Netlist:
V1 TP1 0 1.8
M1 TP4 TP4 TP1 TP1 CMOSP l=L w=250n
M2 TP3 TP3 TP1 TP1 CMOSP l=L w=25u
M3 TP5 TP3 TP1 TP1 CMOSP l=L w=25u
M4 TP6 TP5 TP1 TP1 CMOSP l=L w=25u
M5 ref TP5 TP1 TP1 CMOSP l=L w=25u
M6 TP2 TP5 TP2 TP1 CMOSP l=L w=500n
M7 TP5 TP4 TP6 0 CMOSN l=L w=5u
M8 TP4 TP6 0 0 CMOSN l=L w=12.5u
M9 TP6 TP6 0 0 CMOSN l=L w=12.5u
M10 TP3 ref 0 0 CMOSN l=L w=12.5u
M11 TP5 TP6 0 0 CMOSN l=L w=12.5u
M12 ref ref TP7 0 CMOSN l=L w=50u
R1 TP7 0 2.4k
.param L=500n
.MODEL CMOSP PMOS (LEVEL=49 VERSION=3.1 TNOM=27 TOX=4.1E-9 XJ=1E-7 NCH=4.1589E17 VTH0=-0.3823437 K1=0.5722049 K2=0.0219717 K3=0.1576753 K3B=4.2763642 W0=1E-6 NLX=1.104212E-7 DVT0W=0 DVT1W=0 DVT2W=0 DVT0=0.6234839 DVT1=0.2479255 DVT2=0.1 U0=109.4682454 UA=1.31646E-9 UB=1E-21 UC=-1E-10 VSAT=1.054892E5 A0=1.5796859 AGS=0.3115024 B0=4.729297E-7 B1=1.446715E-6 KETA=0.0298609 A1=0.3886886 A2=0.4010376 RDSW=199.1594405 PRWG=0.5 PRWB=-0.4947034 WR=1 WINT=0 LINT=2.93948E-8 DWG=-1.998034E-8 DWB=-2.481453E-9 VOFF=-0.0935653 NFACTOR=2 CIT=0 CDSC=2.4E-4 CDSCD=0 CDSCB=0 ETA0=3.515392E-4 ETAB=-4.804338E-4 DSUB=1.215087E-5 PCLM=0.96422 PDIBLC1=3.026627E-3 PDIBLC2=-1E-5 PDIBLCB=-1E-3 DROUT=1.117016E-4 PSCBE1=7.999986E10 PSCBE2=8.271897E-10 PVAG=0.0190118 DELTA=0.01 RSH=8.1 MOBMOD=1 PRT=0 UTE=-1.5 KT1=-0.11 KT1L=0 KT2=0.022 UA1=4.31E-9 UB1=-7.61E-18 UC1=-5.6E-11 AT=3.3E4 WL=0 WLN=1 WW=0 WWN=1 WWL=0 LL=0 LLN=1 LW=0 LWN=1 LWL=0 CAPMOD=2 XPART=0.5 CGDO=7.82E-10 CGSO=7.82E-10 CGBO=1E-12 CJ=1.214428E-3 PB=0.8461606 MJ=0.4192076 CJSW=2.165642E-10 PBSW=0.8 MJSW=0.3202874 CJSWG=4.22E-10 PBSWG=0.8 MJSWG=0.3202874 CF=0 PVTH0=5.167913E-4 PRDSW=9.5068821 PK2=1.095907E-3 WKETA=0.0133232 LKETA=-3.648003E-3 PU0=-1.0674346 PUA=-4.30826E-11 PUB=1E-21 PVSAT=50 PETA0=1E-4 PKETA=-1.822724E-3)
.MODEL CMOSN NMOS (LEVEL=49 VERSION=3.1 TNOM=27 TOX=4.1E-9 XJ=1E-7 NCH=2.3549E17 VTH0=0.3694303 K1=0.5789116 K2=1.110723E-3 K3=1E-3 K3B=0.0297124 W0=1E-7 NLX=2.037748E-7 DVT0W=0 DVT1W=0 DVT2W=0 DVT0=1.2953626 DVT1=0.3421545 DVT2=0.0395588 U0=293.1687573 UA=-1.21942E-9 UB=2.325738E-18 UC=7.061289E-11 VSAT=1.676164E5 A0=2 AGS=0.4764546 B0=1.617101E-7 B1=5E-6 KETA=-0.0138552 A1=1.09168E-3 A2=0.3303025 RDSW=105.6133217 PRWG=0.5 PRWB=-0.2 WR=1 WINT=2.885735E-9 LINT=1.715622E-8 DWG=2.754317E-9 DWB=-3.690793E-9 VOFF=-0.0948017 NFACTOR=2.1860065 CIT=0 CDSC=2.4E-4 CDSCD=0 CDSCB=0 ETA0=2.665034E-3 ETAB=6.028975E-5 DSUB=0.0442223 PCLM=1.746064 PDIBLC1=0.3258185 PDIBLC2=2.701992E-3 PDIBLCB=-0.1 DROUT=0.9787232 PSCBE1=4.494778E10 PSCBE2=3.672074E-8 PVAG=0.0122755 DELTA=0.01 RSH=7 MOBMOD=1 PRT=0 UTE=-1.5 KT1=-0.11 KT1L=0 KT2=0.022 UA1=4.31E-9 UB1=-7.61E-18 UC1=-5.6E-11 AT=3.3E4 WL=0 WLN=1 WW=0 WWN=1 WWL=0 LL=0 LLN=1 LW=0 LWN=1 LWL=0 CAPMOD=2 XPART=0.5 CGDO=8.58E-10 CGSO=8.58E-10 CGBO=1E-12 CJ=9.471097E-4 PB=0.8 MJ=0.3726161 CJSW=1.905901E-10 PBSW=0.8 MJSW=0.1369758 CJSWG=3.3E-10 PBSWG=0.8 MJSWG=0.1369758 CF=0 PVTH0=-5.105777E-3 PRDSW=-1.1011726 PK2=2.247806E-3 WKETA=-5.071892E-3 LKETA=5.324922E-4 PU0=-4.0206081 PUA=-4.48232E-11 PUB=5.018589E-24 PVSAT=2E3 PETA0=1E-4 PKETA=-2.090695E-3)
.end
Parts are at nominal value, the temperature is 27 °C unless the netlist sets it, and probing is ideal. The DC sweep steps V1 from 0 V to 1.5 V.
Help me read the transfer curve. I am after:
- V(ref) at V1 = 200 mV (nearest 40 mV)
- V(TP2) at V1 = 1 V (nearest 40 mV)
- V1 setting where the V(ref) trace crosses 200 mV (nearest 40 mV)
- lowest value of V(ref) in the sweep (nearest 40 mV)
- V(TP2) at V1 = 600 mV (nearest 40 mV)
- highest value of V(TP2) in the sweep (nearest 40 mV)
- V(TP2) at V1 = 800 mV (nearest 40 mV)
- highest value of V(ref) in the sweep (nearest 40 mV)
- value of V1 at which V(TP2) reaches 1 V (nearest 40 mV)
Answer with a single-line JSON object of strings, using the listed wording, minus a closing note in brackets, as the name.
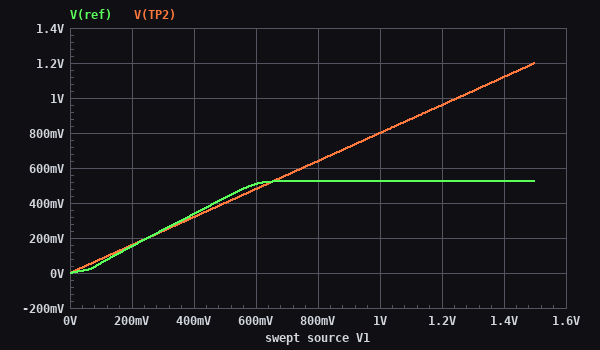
{"V(ref) at V1 = 200 mV": "160 mV", "V(TP2) at V1 = 1 V": "800 mV", "V1 setting where the V(ref) trace crosses 200 mV": "240 mV", "lowest value of V(ref) in the sweep": "0 V", "V(TP2) at V1 = 600 mV": "480 mV", "highest value of V(TP2) in the sweep": "1.20 V", "V(TP2) at V1 = 800 mV": "640 mV", "highest value of V(ref) in the sweep": "520 mV", "value of V1 at which V(TP2) reaches 1 V": "1.24 V"}
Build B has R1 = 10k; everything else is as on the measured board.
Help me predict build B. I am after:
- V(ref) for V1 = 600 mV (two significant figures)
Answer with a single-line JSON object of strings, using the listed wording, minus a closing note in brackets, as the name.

{"V(ref) for V1 = 600 mV": "450 mV"}
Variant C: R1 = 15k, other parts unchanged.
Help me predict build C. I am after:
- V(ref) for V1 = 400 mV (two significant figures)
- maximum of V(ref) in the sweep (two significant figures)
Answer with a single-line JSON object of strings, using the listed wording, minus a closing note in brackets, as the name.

{"V(ref) for V1 = 400 mV": "350 mV", "maximum of V(ref) in the sweep": "430 mV"}
